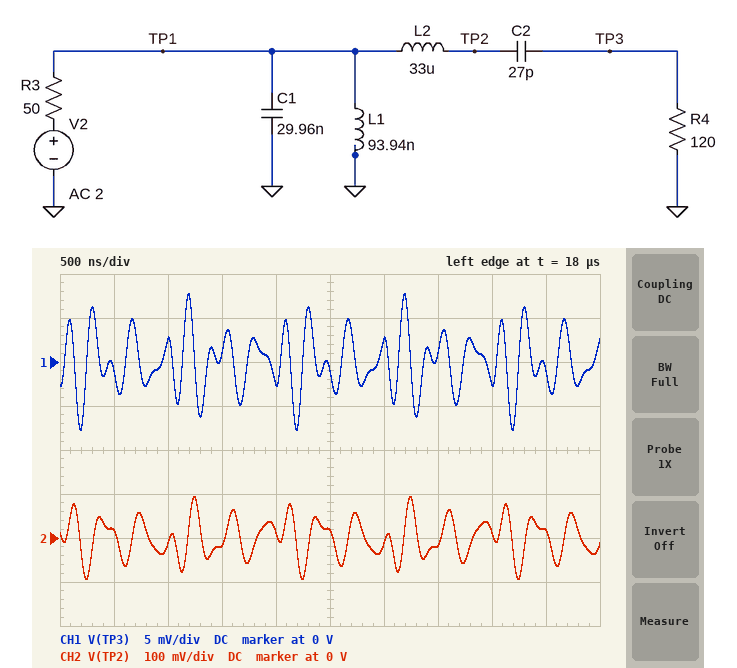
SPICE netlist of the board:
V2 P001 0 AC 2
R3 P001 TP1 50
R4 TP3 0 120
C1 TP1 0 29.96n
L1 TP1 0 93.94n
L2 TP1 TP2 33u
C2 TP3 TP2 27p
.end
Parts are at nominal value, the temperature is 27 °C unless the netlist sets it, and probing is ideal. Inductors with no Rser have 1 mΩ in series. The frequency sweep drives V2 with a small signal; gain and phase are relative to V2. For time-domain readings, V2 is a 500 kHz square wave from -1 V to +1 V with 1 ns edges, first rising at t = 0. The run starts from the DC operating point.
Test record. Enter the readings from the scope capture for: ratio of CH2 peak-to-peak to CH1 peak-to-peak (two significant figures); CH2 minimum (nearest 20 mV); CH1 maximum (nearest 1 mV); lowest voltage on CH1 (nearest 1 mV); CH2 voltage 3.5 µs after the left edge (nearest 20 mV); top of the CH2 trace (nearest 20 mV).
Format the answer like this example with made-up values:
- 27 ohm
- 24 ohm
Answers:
- 12
- -100 mV
- 8 mV
- -8 mV
- -20 mV
- 100 mV
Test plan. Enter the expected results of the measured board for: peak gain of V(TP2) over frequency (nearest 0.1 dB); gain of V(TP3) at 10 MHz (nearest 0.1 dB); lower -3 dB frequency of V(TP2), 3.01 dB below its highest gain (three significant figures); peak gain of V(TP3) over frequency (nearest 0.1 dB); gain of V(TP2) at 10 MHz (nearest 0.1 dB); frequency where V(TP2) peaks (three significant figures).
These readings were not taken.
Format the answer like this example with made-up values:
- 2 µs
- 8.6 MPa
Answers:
- 3.1 dB
- -60.5 dB
- 2.95 MHz
- -21.2 dB
- -46.5 dB
- 3.00 MHz
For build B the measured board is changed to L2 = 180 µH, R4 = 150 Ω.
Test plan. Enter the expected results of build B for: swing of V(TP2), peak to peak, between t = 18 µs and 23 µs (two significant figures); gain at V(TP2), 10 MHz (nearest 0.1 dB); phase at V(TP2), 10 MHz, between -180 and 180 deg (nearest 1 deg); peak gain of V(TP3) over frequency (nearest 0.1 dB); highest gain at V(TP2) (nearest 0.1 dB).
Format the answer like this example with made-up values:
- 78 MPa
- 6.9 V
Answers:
- 280 mV
- -63.6 dB
- 106 deg
- -19.8 dB
- 2.6 dB
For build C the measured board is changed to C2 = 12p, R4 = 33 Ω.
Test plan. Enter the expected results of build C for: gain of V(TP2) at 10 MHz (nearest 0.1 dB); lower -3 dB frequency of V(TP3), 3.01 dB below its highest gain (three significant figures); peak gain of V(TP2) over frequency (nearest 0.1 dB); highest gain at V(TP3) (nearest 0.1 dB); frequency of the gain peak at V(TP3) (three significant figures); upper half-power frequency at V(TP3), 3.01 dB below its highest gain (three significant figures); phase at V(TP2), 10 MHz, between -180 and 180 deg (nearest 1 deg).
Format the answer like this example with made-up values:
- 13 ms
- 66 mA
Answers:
- -33.7 dB
- 7.92 MHz
- 1.2 dB
- -36.2 dB
- 8.00 MHz
- 8.08 MHz
- 95 deg
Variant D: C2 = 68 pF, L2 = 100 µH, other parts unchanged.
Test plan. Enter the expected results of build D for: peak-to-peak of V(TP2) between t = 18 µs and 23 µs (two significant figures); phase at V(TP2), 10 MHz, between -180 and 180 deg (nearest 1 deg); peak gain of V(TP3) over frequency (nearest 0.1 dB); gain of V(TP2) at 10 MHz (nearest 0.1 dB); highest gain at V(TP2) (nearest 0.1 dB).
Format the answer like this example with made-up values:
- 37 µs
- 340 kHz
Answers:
- 130 mV
- 119 deg
- -19.5 dB
- -65.9 dB
- -3.2 dB
